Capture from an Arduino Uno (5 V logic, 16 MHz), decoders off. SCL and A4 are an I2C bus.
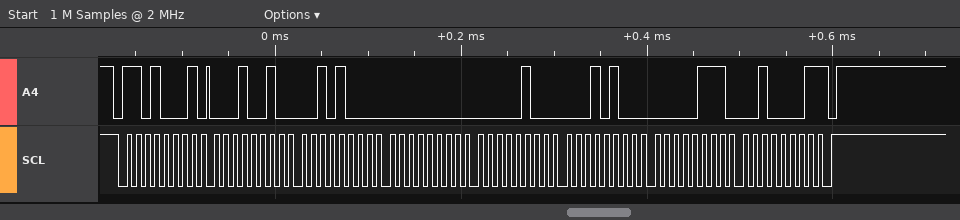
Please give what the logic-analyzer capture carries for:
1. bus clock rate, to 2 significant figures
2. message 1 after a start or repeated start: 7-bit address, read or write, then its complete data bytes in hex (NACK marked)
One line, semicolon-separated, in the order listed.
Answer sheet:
100 kHz; 0x68 read: 12 28 00 04 14 07 21 NACK
